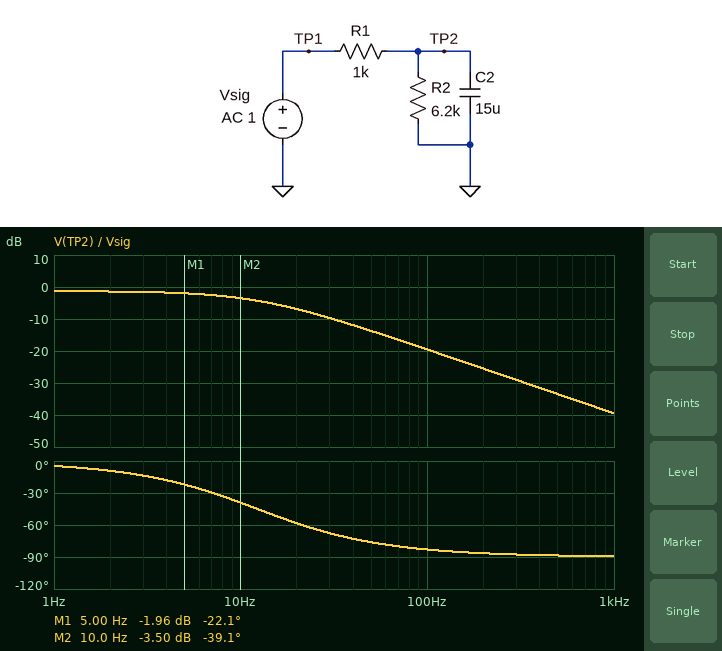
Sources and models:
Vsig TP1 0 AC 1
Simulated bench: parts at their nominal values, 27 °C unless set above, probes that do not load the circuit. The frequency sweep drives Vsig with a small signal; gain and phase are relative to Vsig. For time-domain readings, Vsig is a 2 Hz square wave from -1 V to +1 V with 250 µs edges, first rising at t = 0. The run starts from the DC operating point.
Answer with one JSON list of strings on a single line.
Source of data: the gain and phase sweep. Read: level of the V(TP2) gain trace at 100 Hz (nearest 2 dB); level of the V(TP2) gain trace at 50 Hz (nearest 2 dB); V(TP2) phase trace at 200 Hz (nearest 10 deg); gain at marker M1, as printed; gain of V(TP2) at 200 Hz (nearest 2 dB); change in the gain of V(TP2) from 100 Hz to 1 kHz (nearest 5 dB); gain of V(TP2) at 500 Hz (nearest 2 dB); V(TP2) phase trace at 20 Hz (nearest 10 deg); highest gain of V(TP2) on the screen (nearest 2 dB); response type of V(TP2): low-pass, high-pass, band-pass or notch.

["-20 dB", "-14 dB", "-90 deg", "-1.96 dB", "-26 dB", "-20 dB", "-34 dB", "-60 deg", "-2 dB", "low-pass"]
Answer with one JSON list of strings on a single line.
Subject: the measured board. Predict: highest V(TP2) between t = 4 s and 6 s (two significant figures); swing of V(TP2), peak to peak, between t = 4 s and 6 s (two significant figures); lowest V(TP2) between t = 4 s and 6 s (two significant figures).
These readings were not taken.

["860 mV", "1.7 V", "-860 mV"]
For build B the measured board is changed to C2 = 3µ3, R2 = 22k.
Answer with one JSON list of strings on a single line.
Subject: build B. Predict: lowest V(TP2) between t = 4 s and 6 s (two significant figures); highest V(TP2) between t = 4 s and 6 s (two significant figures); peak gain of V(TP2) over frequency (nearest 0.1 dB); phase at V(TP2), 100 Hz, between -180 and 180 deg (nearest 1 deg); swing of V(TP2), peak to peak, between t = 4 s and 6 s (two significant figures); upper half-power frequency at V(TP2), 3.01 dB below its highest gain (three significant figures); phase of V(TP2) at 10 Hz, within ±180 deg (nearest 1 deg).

["-960 mV", "960 mV", "-0.4 dB", "-63 deg", "1.9 V", "50.4 Hz", "-11 deg"]
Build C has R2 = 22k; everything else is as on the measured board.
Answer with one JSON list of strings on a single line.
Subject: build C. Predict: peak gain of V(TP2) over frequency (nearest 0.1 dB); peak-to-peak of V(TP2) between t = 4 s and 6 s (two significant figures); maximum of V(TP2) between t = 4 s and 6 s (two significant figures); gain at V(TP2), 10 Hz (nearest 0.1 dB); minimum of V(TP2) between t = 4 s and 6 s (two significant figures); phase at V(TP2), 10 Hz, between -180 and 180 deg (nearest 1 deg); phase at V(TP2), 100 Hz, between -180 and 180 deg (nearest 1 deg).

["-0.4 dB", "1.9 V", "960 mV", "-3.0 dB", "-960 mV", "-42 deg", "-84 deg"]
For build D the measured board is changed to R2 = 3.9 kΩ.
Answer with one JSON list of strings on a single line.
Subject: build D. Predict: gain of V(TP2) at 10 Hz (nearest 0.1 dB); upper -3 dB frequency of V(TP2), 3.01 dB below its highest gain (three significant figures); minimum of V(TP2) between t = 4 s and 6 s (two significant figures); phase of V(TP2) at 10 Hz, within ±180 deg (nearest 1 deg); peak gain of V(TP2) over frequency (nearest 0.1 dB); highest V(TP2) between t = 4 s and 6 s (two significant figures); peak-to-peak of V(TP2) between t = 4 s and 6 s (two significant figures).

["-3.9 dB", "13.3 Hz", "-800 mV", "-37 deg", "-2.0 dB", "800 mV", "1.6 V"]
